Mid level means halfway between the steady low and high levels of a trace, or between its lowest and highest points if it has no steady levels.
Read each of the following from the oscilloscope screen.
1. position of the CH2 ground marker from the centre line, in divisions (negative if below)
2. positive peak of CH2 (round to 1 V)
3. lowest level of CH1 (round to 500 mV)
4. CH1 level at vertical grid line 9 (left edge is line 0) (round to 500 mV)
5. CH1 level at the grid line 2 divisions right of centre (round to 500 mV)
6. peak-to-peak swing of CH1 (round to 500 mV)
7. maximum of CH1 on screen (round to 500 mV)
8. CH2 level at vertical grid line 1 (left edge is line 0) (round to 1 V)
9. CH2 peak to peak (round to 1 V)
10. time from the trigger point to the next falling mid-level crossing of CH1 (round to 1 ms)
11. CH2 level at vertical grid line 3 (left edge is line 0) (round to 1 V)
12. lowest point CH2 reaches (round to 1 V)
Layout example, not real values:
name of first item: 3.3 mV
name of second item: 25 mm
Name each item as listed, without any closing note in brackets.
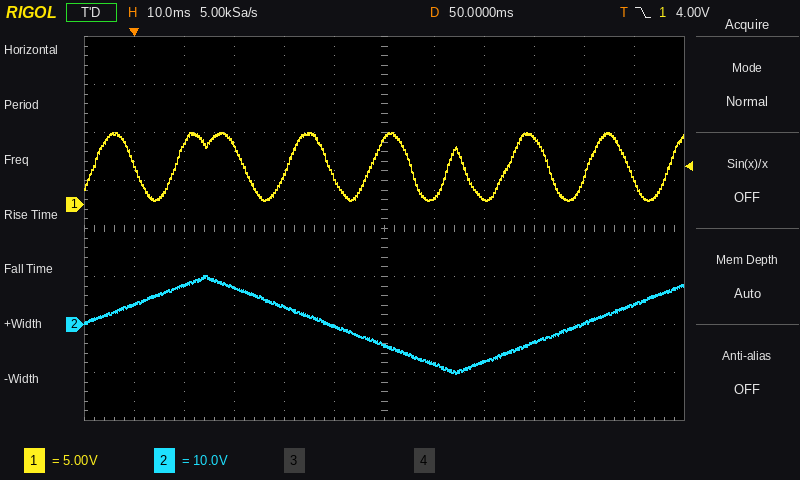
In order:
position of the CH2 ground marker from the centre line, in divisions: -2.0 div
positive peak of CH2: 10 V
lowest level of CH1: 500 mV
CH1 level at vertical grid line 9 (left edge is line 0): 7.0 V
CH1 level at the grid line 2 divisions right of centre: 500 mV
peak-to-peak swing of CH1: 7.0 V
maximum of CH1 on screen: 7.5 V
CH2 level at vertical grid line 1 (left edge is line 0): 4 V
CH2 peak to peak: 20 V
time from the trigger point to the next falling mid-level crossing of CH1: 22 ms
CH2 level at vertical grid line 3 (left edge is line 0): 8 V
lowest point CH2 reaches: -10 V
